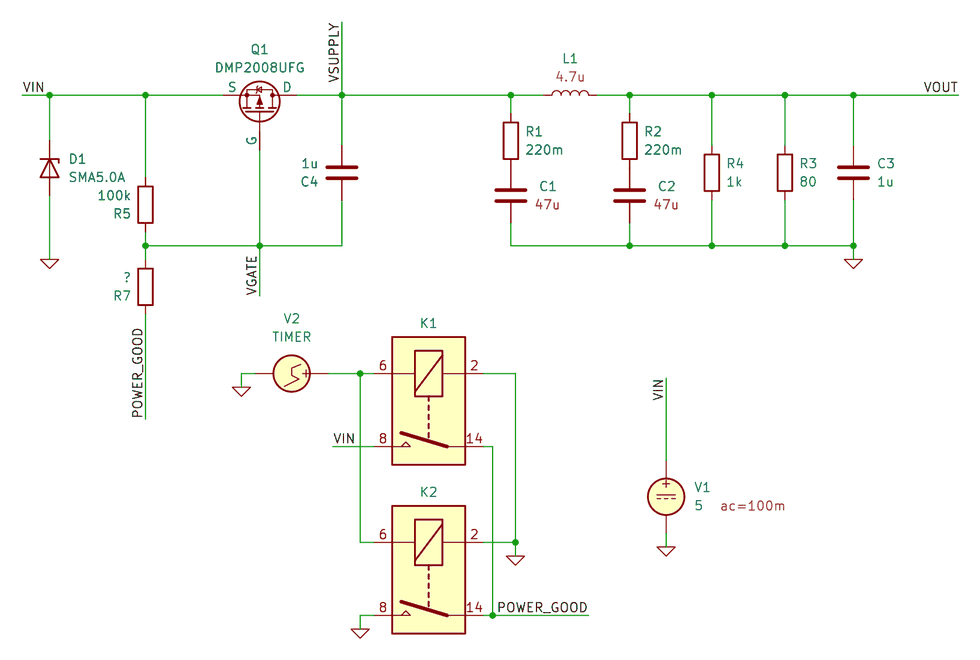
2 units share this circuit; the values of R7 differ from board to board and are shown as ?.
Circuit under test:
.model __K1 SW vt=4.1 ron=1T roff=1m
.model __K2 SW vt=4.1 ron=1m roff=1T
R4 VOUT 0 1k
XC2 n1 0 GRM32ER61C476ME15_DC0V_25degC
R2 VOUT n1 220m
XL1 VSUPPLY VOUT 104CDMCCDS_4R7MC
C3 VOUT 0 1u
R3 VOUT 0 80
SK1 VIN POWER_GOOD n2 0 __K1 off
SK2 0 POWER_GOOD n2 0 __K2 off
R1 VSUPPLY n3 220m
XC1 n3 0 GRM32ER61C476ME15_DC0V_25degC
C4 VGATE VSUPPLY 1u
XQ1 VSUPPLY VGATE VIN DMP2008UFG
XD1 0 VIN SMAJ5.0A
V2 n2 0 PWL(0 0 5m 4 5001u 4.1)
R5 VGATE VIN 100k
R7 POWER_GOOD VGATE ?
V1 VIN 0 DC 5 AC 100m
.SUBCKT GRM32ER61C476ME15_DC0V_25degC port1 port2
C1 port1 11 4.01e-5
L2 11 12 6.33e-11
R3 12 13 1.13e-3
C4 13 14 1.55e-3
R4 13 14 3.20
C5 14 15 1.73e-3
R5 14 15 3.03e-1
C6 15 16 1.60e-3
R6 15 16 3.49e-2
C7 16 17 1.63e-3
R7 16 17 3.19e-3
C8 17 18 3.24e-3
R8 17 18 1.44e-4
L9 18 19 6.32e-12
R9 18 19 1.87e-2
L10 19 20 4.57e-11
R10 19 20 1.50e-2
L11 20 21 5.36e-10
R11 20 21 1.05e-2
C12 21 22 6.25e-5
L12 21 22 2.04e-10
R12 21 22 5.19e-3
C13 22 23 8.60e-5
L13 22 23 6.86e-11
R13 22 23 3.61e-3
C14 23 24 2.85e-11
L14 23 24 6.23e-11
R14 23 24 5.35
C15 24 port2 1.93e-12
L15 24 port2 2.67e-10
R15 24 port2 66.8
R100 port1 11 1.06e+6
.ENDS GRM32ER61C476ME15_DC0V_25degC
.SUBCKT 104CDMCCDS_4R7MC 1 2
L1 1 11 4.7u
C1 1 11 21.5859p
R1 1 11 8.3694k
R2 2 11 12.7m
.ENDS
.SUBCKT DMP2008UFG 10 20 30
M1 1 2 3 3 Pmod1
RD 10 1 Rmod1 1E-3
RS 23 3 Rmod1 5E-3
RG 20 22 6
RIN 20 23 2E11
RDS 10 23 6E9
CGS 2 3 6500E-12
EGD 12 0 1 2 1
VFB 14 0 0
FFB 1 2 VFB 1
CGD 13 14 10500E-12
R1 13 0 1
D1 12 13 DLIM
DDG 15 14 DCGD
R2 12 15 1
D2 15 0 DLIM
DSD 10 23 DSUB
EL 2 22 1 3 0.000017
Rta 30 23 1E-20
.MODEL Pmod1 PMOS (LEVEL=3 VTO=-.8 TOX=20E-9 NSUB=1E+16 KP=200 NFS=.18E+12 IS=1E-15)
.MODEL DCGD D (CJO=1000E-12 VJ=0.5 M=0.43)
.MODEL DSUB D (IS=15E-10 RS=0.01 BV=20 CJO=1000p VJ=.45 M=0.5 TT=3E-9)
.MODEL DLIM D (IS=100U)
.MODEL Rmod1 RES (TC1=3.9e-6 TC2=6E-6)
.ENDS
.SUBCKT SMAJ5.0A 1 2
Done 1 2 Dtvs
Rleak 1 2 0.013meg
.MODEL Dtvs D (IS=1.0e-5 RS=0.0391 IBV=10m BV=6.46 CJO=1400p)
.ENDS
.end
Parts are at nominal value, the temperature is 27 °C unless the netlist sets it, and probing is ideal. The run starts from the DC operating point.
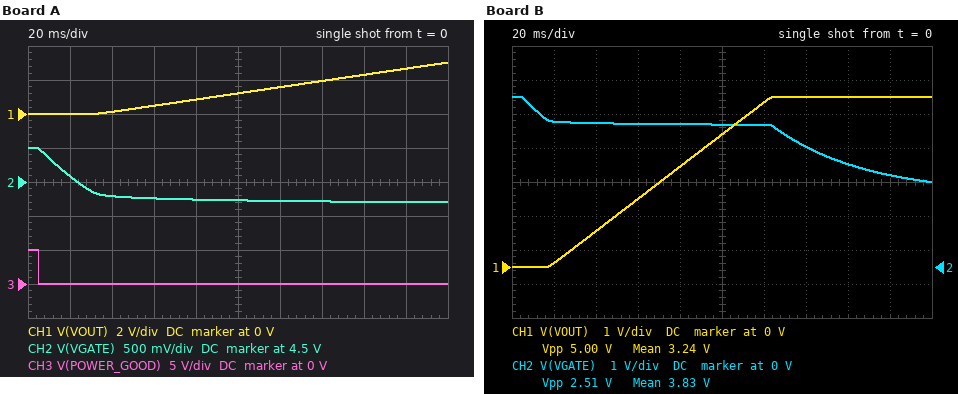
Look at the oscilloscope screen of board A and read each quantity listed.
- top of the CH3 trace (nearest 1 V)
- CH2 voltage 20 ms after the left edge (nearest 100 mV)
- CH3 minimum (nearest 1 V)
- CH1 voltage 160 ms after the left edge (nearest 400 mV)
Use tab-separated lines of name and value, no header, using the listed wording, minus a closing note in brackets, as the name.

top of the CH3 trace	5 V
CH2 voltage 20 ms after the left edge	4.6 V
CH3 minimum	0 V
CH1 voltage 160 ms after the left edge	2.4 V
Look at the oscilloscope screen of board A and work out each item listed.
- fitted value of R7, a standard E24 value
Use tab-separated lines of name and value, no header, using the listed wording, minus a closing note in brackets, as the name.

fitted value of R7, a standard E24 value	160 kΩ
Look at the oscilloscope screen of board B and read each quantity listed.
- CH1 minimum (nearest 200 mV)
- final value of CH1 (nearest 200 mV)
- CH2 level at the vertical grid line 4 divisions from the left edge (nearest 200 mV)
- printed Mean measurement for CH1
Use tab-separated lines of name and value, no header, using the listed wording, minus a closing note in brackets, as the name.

CH1 minimum	0 V
final value of CH1	5.0 V
CH2 level at the vertical grid line 4 divisions from the left edge	4.2 V
printed Mean measurement for CH1	3.24 V
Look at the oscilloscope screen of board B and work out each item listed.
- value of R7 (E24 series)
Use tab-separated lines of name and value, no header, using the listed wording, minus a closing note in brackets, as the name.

value of R7	75 kΩ
